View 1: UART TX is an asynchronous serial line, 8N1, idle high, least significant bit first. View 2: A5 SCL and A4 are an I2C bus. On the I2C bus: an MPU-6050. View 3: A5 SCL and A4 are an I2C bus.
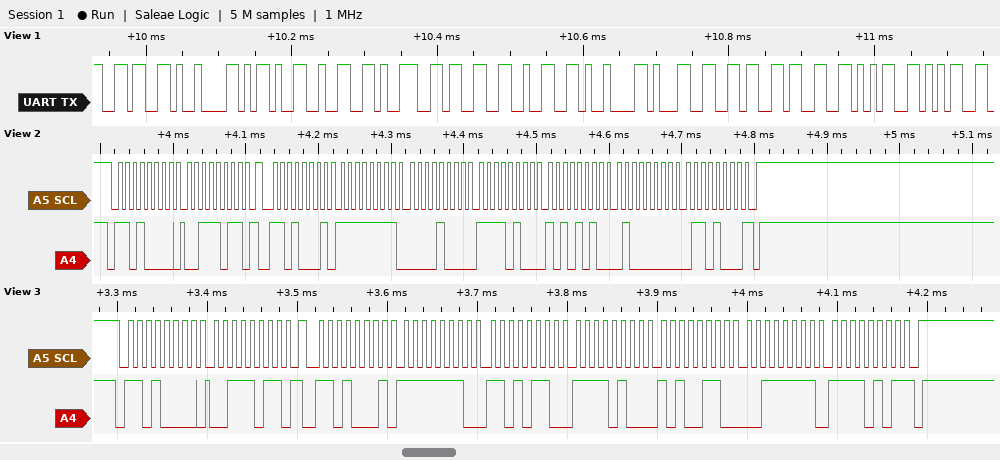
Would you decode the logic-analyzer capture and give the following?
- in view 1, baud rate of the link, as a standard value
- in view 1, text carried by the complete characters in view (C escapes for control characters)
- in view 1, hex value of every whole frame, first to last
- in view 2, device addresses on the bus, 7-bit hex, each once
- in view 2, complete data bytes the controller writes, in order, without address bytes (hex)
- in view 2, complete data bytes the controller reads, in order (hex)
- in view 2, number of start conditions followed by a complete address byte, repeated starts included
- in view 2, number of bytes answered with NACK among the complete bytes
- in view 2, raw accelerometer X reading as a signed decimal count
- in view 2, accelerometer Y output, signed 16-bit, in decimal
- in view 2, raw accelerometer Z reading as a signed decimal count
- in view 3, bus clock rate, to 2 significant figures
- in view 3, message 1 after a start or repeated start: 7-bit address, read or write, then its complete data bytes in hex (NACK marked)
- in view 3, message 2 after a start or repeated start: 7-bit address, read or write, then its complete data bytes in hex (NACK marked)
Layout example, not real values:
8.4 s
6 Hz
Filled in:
115200 baud
"6\t-2932\t16355"
0x36 0x09 0x2D 0x32 0x39 0x33 0x32 0x09 0x31 0x36 0x33 0x35 0x35
0x68
3B
FF 08 F4 AA 40 68
2
1
-248
-2902
16488
100 kHz
0x68 write: 3B
0x68 read: FE D6 F4 A6 3F F5 NACK
